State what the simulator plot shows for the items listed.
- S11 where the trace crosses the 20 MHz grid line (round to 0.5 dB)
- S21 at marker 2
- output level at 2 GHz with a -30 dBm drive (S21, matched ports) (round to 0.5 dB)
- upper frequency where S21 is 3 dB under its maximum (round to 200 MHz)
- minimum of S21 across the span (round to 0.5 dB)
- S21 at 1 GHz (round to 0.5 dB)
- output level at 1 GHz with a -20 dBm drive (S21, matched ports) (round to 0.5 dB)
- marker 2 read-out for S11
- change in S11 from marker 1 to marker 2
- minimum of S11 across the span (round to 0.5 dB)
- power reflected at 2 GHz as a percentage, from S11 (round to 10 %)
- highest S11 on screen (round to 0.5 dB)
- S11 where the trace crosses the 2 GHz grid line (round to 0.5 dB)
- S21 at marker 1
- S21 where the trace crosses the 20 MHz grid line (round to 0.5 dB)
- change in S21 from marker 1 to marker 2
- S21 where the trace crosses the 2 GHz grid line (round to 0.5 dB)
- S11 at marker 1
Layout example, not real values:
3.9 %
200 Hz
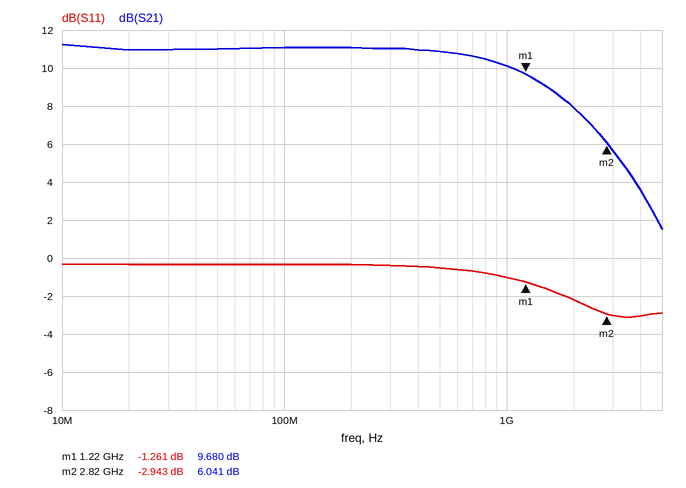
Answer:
-0.5 dB
6.041 dB
-22.0 dBm
1.8 GHz
1.5 dB
10.0 dB
-10.0 dBm
-2.943 dB
-1.682 dB
-3.0 dB
60 %
-0.5 dB
-2.0 dB
9.680 dB
11.0 dB
-3.639 dB
8.0 dB
-1.261 dB
